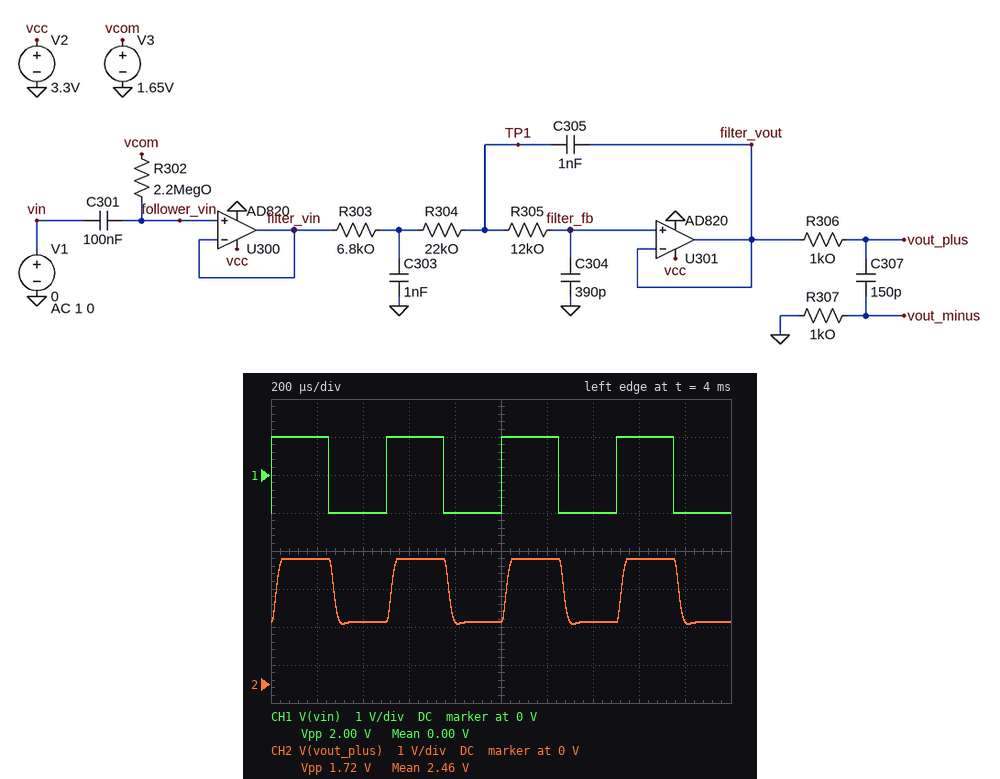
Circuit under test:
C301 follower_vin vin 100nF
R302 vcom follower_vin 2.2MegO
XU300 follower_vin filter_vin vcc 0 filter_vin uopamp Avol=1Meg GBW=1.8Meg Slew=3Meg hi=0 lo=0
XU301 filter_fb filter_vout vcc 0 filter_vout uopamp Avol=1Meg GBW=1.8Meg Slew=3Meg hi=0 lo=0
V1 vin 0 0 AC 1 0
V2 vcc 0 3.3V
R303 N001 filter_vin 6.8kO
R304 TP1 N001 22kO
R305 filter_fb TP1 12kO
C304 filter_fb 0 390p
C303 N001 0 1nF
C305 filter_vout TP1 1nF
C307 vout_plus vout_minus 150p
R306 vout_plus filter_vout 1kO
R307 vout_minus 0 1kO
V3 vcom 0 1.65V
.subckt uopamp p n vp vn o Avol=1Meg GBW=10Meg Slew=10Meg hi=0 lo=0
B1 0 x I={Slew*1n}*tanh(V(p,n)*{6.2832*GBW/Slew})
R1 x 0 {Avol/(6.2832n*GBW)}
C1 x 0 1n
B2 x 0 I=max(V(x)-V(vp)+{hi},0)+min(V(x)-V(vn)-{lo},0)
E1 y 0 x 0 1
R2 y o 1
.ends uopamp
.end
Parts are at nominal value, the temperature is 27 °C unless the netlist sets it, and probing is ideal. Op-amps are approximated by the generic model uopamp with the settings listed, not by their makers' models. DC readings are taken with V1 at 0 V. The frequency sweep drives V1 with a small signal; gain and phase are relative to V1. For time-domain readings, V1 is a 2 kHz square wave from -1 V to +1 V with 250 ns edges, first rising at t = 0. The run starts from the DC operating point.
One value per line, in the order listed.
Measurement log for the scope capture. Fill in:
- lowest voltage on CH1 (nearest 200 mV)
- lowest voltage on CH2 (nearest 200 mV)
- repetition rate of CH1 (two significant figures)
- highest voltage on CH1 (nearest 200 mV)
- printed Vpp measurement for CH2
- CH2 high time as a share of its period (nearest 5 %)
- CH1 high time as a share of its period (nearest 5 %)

-1.0 V
1.6 V
2.0 kHz
1.0 V
1.72 V
50 %
50 %
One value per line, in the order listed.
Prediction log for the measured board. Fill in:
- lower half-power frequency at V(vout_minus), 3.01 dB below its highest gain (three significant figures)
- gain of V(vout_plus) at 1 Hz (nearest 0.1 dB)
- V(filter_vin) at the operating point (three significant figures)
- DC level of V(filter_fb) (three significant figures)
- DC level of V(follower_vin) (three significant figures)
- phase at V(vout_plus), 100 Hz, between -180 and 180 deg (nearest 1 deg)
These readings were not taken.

6.34 kHz
-1.8 dB
1.65 V
1.65 V
1.65 V
0 deg
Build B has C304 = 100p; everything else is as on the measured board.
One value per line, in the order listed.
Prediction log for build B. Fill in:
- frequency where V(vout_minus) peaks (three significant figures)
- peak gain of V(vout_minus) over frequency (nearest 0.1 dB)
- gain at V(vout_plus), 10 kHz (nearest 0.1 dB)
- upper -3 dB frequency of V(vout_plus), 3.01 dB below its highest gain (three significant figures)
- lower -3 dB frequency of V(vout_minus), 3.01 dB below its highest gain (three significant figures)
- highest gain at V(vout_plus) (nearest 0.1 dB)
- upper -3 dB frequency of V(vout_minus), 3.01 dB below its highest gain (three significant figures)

25.9 kHz
-33.2 dB
0.1 dB
30.1 kHz
16.1 kHz
0.2 dB
36.9 kHz
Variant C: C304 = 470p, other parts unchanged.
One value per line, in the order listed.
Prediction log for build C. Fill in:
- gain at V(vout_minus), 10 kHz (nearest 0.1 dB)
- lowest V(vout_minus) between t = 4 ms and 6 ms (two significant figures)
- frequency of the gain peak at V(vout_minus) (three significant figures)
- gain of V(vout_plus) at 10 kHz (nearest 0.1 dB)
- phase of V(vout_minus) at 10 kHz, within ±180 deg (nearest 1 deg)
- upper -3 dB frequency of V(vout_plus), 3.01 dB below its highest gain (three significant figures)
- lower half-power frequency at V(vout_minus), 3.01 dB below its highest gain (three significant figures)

-43.6 dB
-7.6 mV
11.4 kHz
-3.1 dB
-5 deg
9.93 kHz
5.52 kHz
